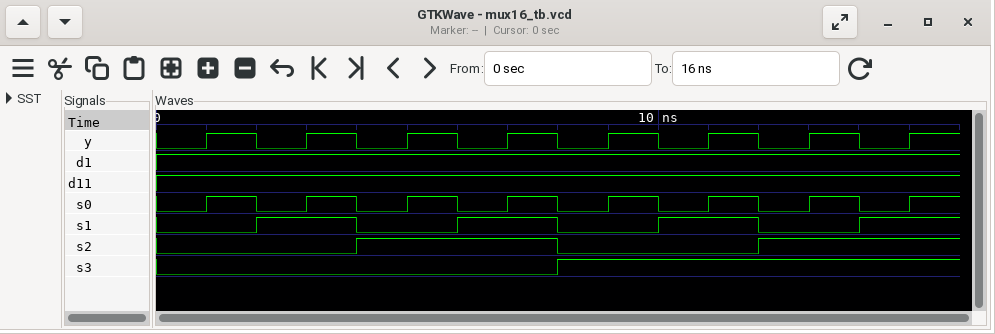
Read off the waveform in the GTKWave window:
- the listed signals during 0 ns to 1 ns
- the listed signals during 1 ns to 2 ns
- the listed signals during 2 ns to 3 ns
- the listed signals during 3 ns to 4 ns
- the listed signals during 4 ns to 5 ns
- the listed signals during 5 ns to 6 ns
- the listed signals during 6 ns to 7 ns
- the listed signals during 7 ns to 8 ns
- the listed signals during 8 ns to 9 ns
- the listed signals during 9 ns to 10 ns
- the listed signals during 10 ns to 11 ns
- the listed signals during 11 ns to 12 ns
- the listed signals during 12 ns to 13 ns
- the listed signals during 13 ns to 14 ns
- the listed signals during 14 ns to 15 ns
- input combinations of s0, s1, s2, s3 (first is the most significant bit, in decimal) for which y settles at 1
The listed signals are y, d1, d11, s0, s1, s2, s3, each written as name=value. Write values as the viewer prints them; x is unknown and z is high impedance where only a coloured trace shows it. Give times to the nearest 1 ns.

y=0, d1=1, d11=1, s0=0, s1=0, s2=0, s3=0
y=1, d1=1, d11=1, s0=1, s1=0, s2=0, s3=0
y=0, d1=1, d11=1, s0=0, s1=1, s2=0, s3=0
y=1, d1=1, d11=1, s0=1, s1=1, s2=0, s3=0
y=0, d1=1, d11=1, s0=0, s1=0, s2=1, s3=0
y=1, d1=1, d11=1, s0=1, s1=0, s2=1, s3=0
y=0, d1=1, d11=1, s0=0, s1=1, s2=1, s3=0
y=1, d1=1, d11=1, s0=1, s1=1, s2=1, s3=0
y=0, d1=1, d11=1, s0=0, s1=0, s2=0, s3=1
y=1, d1=1, d11=1, s0=1, s1=0, s2=0, s3=1
y=0, d1=1, d11=1, s0=0, s1=1, s2=0, s3=1
y=1, d1=1, d11=1, s0=1, s1=1, s2=0, s3=1
y=0, d1=1, d11=1, s0=0, s1=0, s2=1, s3=1
y=1, d1=1, d11=1, s0=1, s1=0, s2=1, s3=1
y=0, d1=1, d11=1, s0=0, s1=1, s2=1, s3=1
8, 9, 10, 11, 12, 13, 14, 15
